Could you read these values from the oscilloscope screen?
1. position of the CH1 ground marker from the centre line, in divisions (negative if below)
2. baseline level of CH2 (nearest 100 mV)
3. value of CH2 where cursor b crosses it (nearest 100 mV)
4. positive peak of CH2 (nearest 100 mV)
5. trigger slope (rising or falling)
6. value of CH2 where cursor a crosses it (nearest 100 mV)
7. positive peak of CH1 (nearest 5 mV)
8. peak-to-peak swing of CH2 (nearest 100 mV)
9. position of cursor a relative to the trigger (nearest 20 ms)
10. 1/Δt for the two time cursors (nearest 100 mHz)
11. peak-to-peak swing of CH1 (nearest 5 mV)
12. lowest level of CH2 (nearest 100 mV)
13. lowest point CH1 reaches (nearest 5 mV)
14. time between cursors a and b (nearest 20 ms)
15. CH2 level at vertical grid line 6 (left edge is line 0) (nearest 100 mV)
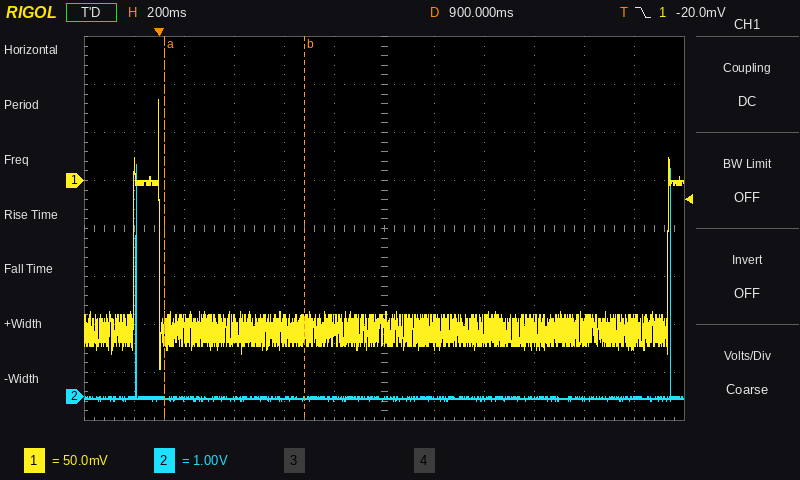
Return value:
+1.0 div
0.0 V
0.0 V
4.8 V
falling
0.0 V
85 mV
4.9 V
+20 ms
1.8 Hz
280 mV
-100 mV
-195 mV
560 ms
0.0 V
